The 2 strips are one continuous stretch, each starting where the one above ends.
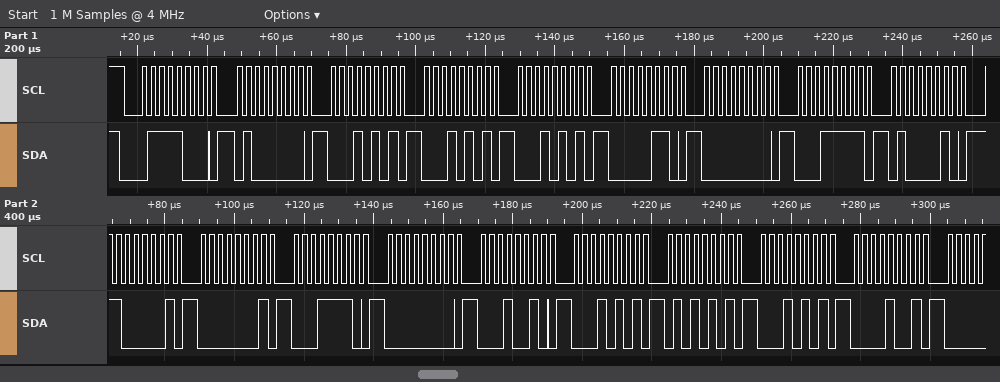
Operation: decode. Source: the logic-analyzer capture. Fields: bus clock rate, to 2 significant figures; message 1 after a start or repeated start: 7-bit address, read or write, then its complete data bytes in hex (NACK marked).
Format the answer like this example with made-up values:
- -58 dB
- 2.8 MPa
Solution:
- 400 kHz
- 0x3C write: 40 15 15 15 06 00 1F 42 C1 01 1E 00 12 15 55 15 09
